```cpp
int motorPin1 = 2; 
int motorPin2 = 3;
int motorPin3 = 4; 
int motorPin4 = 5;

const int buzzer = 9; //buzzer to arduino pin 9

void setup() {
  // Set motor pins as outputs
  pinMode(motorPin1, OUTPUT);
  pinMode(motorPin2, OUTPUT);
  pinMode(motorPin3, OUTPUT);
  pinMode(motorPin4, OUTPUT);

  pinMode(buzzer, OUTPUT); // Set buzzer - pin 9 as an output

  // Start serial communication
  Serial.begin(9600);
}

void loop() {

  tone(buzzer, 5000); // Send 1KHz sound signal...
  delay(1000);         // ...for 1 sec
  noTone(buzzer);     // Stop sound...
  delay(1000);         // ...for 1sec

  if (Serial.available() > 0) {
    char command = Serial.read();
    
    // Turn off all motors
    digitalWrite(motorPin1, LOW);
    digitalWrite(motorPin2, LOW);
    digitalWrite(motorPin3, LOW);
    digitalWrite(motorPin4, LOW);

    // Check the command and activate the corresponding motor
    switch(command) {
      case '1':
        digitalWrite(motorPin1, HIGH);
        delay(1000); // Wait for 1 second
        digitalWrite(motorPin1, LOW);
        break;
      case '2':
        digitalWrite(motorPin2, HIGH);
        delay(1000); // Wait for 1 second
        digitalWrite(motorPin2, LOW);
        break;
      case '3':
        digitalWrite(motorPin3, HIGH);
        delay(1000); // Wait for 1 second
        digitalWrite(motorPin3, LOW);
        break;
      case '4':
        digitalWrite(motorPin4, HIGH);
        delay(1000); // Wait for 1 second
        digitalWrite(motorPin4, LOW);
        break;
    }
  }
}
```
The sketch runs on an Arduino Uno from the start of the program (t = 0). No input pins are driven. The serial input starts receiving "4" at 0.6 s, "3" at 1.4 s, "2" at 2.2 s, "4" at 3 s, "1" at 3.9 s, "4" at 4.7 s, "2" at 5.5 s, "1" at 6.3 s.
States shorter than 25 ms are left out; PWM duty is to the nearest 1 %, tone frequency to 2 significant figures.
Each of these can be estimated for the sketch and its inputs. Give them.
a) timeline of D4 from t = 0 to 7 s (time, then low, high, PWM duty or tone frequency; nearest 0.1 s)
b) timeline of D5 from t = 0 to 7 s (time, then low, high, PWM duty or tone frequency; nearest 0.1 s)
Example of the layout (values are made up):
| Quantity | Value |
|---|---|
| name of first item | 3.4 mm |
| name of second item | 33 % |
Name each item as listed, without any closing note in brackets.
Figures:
| Quantity | Value |
|---|---|
| timeline of D4 from t = 0 to 7 s | 0 s low; 5 s high; 6 s low |
| timeline of D5 from t = 0 to 7 s | 0 s low; 2 s high; 3 s low |
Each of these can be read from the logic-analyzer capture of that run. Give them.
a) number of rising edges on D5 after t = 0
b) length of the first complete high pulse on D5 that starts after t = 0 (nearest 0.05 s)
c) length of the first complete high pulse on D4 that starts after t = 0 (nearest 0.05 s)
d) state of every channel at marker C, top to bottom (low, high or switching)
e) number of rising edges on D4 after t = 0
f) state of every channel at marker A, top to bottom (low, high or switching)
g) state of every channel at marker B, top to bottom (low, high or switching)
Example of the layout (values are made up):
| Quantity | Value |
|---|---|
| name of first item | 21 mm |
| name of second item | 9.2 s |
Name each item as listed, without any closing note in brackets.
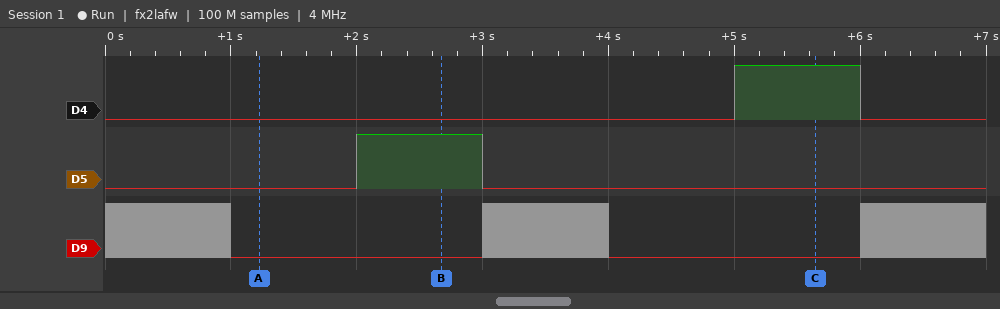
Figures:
| Quantity | Value |
|---|---|
| number of rising edges on D5 after t = 0 | 1 |
| length of the first complete high pulse on D5 that starts after t = 0 | 1.00 s |
| length of the first complete high pulse on D4 that starts after t = 0 | 1.00 s |
| state of every channel at marker C, top to bottom | D4 high, D5 low, D9 low |
| number of rising edges on D4 after t = 0 | 1 |
| state of every channel at marker A, top to bottom | D4 low, D5 low, D9 low |
| state of every channel at marker B, top to bottom | D4 low, D5 high, D9 low |
